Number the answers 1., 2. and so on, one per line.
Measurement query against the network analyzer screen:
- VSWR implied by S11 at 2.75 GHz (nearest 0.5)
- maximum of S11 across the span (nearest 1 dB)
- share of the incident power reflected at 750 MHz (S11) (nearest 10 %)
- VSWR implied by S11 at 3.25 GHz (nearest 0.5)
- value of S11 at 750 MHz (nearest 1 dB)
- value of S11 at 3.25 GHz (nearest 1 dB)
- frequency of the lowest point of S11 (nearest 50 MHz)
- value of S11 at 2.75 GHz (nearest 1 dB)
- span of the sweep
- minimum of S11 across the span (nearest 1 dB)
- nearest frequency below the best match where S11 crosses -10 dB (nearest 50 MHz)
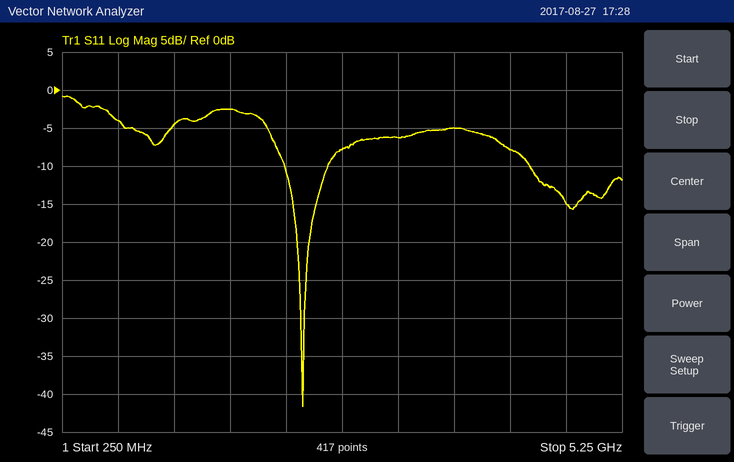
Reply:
1. 2.5
2. -1 dB
3. 40 %
4. 3.0
5. -4 dB
6. -6 dB
7. 2.40 GHz
8. -8 dB
9. 5 GHz
10. -42 dB
11. 2.25 GHz
